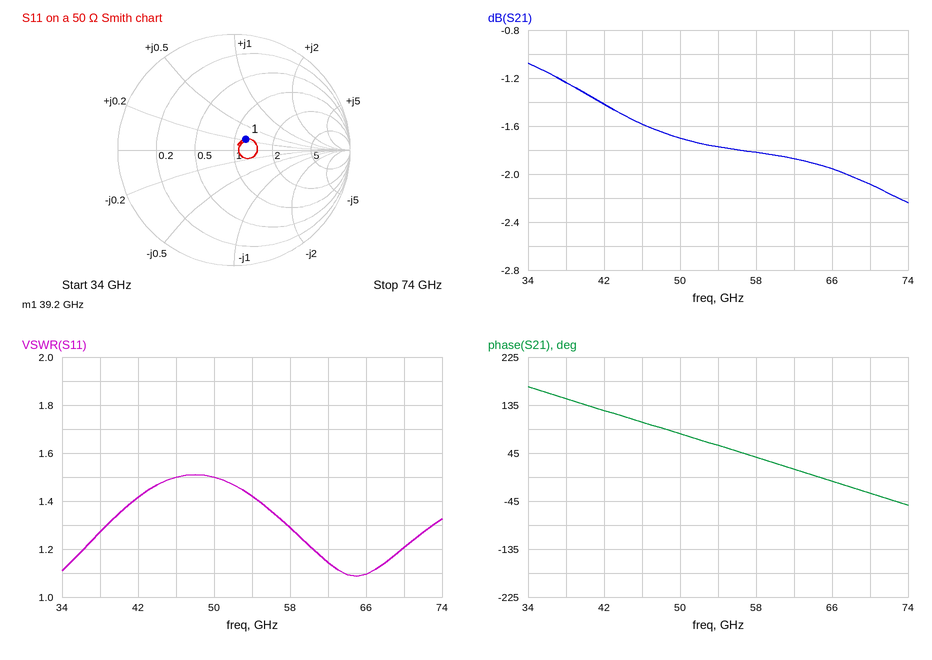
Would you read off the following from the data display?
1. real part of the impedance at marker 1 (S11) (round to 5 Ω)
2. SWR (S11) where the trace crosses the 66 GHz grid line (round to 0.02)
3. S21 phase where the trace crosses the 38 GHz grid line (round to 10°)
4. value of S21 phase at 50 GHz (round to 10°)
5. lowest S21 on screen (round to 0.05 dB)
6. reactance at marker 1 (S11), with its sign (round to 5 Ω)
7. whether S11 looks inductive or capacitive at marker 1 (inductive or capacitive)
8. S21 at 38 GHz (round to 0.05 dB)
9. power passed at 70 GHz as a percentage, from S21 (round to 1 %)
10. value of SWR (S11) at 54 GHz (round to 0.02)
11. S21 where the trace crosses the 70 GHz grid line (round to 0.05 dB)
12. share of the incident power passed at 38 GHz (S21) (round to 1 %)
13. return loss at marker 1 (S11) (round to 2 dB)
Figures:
60 Ω
1.10
150°
80°
-2.25 dB
+10 Ω
inductive
-1.25 dB
62 %
1.42
-2.10 dB
75 %
18 dB
